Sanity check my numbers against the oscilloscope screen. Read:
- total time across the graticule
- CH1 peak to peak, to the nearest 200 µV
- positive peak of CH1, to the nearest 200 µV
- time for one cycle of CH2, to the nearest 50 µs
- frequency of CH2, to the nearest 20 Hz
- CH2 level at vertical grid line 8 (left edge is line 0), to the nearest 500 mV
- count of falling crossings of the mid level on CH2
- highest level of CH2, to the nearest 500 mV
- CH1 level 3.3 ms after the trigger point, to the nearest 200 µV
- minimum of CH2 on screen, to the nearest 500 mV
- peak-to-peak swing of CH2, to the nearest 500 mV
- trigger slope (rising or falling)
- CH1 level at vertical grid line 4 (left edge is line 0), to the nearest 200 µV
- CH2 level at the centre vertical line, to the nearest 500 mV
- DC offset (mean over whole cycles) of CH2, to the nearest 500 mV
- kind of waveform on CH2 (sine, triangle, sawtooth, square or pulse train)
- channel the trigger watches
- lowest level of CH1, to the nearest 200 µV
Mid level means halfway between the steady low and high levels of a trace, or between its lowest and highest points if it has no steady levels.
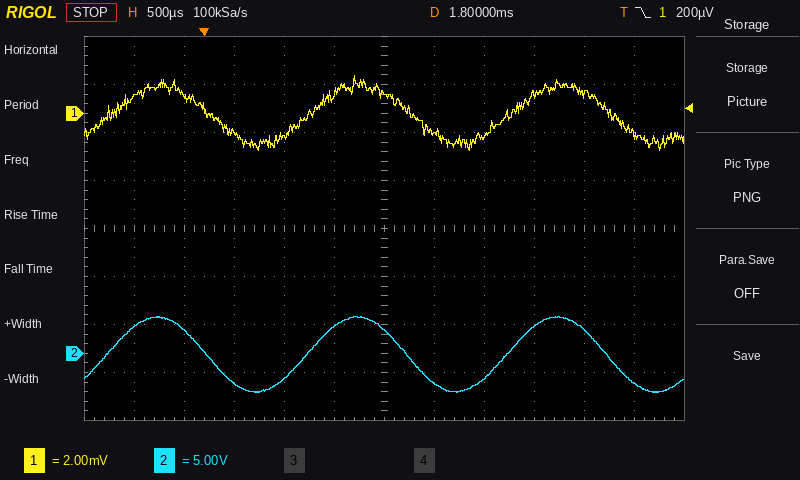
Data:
6 ms
3.2 mV
1.6 mV
2.00 ms
500 Hz
-2.5 V
3
4.0 V
800 µV
-4.0 V
8.0 V
falling
-1.0 mV
2.5 V
0.0 V
sine
CH1
-1.6 mV
